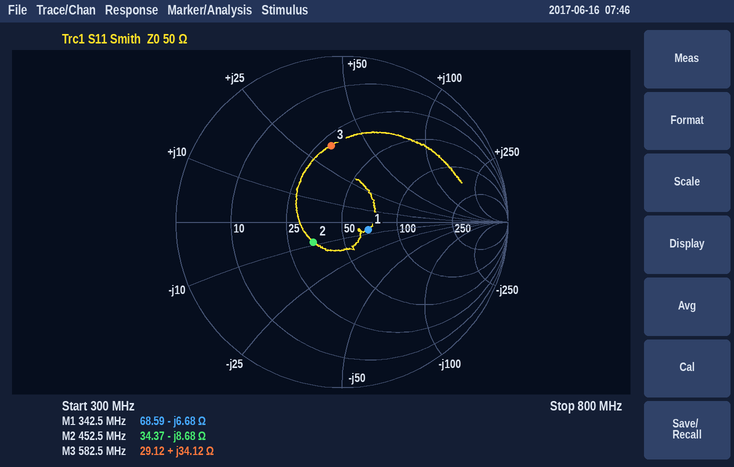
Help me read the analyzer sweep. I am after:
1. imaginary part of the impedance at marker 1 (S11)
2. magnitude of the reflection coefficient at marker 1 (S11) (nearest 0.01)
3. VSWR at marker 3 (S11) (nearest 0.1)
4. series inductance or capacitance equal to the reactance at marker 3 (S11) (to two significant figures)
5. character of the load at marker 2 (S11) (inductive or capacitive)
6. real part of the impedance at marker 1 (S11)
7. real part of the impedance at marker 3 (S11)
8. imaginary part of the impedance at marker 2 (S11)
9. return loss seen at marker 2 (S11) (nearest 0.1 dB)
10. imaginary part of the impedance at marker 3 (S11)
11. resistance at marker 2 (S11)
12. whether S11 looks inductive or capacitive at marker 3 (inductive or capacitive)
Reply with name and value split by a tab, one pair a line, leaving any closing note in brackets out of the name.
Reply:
imaginary part of the impedance at marker 1	-6.68 Ω
magnitude of the reflection coefficient at marker 1 (S11)	0.17
VSWR at marker 3 (S11)	2.7
series inductance or capacitance equal to the reactance at marker 3 (S11)	9.3 nH
character of the load at marker 2 (S11)	capacitive
real part of the impedance at marker 1	68.59 Ω
real part of the impedance at marker 3	29.12 Ω
imaginary part of the impedance at marker 2	-8.68 Ω
return loss seen at marker 2 (S11)	13.5 dB
imaginary part of the impedance at marker 3	+34.12 Ω
resistance at marker 2	34.37 Ω
whether S11 looks inductive or capacitive at marker 3	inductive
